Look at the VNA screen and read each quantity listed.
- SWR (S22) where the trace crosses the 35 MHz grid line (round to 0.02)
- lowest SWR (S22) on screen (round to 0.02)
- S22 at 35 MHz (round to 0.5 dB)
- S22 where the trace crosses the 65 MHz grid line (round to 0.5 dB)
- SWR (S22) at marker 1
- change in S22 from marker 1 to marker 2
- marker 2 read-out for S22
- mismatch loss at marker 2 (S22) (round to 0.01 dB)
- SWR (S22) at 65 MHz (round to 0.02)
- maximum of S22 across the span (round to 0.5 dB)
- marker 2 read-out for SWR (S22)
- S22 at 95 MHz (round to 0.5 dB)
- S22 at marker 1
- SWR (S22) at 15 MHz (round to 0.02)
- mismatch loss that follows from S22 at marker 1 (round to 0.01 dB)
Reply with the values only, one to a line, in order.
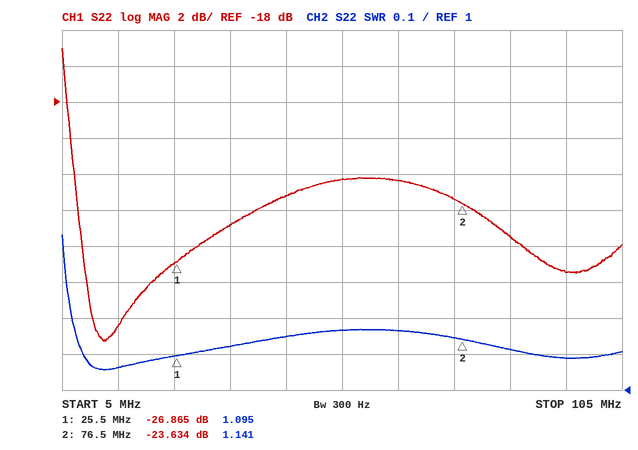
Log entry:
1.12
1.06
-25.0 dB
-22.5 dB
1.095
3.231 dB
-23.634 dB
0.02 dB
1.16
-15.0 dB
1.141
-27.5 dB
-26.865 dB
1.06
0.01 dB
